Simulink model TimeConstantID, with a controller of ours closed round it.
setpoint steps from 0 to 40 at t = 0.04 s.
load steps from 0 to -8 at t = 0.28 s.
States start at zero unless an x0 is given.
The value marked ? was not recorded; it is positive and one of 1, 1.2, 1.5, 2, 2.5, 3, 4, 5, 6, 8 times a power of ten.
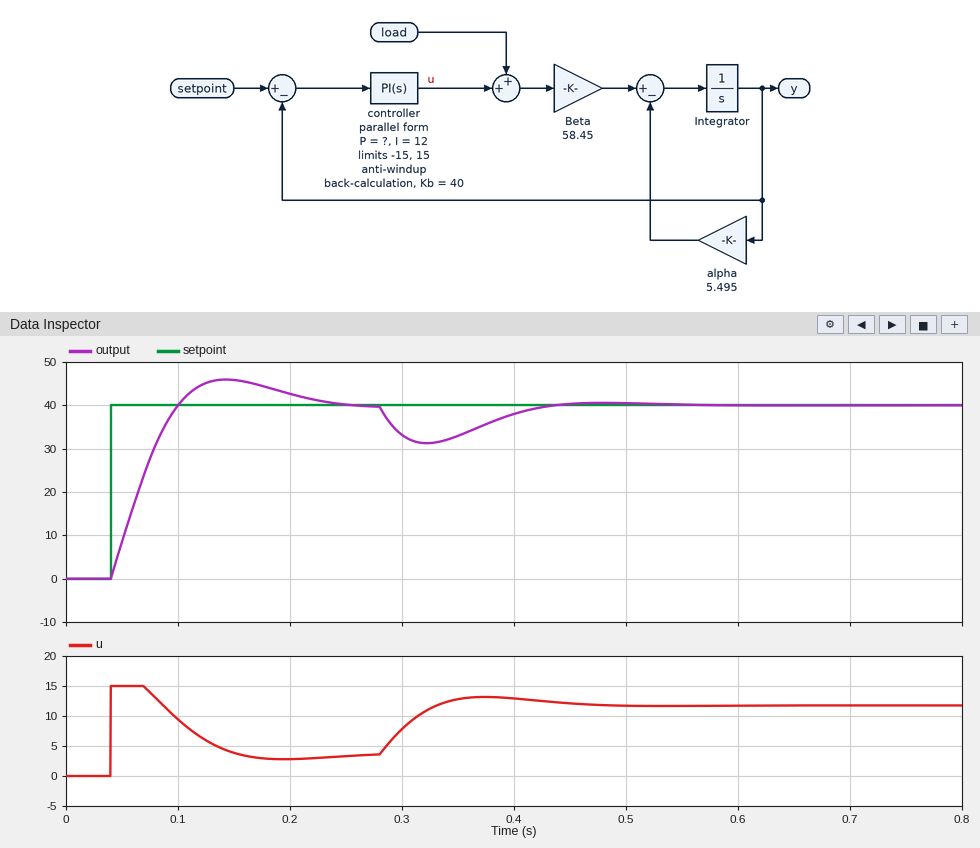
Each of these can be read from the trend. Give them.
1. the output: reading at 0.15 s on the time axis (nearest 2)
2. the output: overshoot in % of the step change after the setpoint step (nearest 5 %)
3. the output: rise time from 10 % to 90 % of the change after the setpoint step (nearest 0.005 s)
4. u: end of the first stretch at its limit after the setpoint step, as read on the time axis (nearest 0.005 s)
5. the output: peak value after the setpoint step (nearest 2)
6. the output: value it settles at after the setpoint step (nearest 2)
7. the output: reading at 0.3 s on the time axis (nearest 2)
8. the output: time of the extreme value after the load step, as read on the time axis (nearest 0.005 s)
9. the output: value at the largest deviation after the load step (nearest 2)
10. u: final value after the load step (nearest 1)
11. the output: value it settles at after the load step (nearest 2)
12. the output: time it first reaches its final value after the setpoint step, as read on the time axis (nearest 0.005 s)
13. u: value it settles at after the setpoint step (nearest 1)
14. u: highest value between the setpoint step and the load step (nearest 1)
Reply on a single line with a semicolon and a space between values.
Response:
46; 15 %; 0.045 s; 0.070 s; 46; 40; 34; 0.320 s; 32; 12; 40; 0.100 s; 4; 15
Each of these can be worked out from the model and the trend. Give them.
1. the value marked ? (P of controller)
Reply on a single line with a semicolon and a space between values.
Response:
0.5
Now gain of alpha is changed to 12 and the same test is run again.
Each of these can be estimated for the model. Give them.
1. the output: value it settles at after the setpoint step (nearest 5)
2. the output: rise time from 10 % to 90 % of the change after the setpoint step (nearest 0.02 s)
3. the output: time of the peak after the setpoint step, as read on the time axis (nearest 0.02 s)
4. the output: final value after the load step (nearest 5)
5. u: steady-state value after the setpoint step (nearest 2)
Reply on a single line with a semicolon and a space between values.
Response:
40; 0.06 s; 0.16 s; 35; 8
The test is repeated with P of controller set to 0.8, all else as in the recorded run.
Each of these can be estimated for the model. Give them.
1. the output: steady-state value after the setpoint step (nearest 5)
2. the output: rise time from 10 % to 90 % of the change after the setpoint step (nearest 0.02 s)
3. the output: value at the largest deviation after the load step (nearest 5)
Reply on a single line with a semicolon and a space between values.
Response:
40; 0.06 s; 35
